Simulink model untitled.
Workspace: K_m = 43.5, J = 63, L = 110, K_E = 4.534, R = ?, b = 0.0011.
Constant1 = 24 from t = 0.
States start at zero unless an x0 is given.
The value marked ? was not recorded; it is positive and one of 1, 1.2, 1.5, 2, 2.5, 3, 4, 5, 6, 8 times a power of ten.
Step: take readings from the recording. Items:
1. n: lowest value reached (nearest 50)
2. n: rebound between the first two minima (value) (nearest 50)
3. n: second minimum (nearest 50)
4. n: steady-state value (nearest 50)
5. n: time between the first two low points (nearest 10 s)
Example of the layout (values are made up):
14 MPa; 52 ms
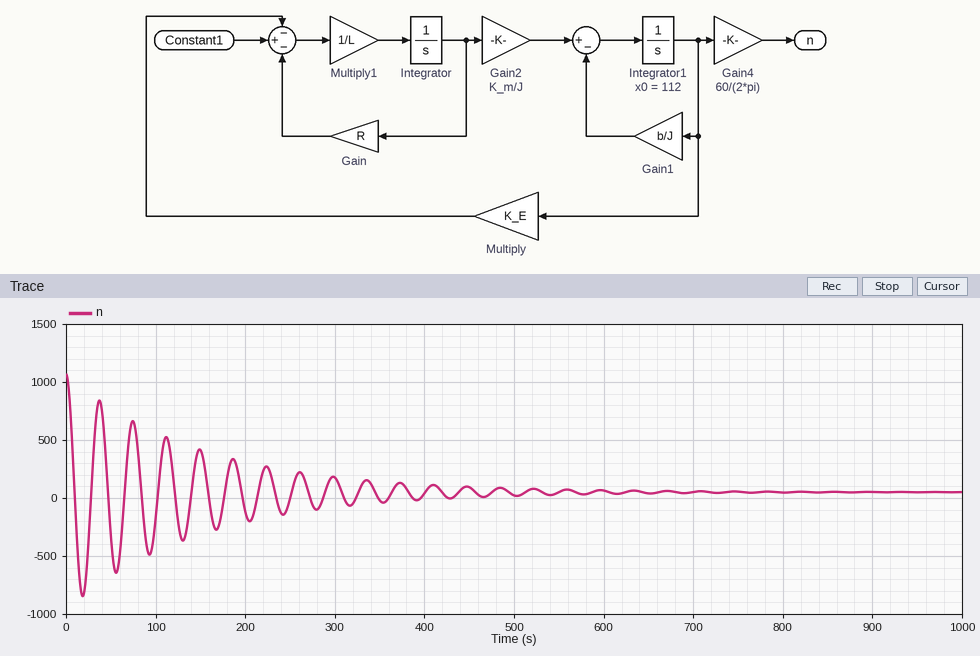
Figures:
-850; 850; -650; 50; 40 s
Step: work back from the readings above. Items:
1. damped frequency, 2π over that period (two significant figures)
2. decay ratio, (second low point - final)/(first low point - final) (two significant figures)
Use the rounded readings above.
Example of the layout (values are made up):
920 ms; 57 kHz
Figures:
0.16 rad/s; 0.78
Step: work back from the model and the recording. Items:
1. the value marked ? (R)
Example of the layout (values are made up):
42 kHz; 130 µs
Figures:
1.5
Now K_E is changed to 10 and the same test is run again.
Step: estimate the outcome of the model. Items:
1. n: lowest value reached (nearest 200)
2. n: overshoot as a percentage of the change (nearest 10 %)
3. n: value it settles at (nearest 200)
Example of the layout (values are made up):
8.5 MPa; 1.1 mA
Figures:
-1000; 90 %; 0
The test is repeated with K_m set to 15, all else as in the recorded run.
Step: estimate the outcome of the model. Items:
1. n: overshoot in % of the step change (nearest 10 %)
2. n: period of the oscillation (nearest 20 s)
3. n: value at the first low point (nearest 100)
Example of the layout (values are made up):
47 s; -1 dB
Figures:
80 %; 60 s; -800
